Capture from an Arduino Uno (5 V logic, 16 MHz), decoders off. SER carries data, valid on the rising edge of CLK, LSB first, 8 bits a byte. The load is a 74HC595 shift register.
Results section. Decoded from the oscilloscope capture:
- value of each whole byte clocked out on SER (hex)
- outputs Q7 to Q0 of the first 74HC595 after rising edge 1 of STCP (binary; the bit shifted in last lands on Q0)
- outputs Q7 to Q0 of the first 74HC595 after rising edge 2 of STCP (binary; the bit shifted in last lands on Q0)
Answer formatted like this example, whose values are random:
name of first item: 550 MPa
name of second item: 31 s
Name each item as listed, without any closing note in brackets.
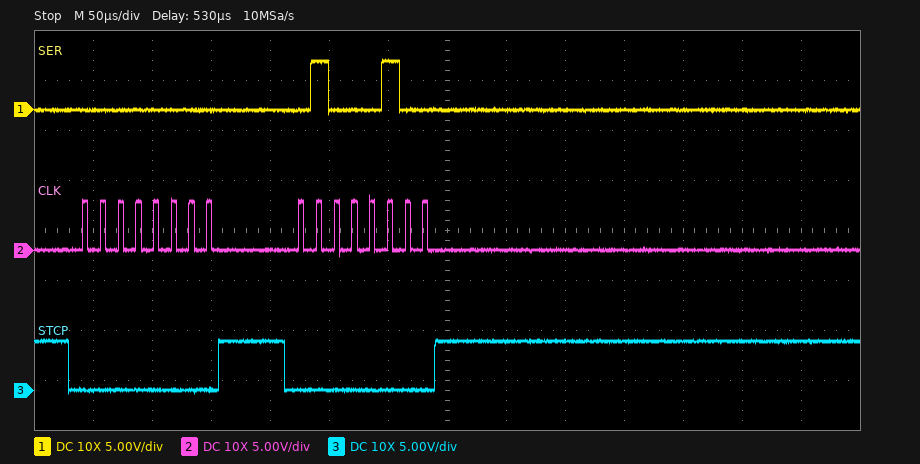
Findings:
value of each whole byte clocked out on SER: 00 22
outputs Q7 to Q0 of the first 74HC595 after rising edge 1 of STCP: 00000000
outputs Q7 to Q0 of the first 74HC595 after rising edge 2 of STCP: 01000100
